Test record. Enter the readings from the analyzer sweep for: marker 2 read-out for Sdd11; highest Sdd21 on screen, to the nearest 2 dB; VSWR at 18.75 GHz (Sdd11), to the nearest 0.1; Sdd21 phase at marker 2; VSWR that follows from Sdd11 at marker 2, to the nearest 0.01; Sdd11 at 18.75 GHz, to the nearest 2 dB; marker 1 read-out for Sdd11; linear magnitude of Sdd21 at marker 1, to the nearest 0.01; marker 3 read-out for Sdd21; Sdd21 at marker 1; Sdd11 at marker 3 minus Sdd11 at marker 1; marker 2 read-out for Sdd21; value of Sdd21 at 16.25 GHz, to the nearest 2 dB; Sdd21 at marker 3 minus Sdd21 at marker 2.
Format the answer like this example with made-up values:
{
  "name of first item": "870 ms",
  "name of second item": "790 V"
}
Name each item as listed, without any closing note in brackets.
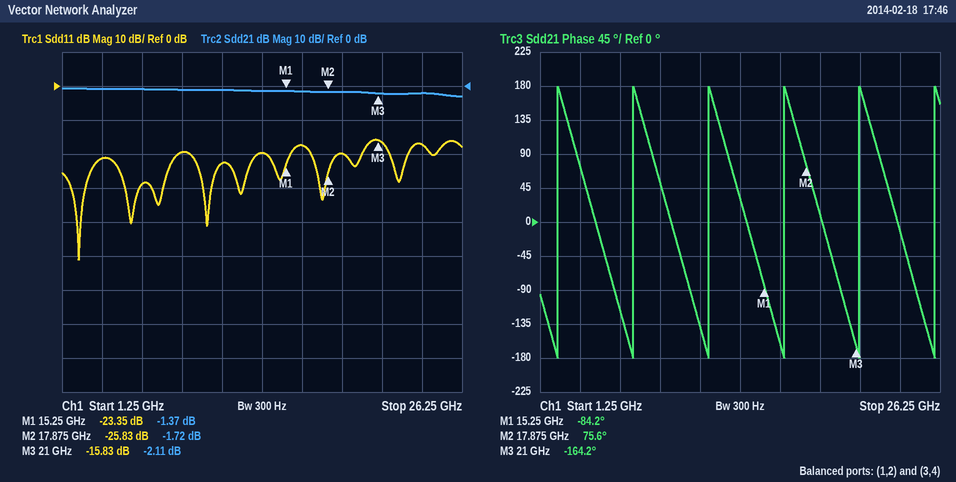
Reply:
{
  "marker 2 read-out for Sdd11": "-25.83 dB",
  "highest Sdd21 on screen, to the nearest 2 dB": "0 dB",
  "VSWR at 18.75 GHz (Sdd11), to the nearest 0.1": "1.2",
  "Sdd21 phase at marker 2": "75.6°",
  "VSWR that follows from Sdd11 at marker 2, to the nearest 0.01": "1.11",
  "Sdd11 at 18.75 GHz, to the nearest 2 dB": "-20 dB",
  "marker 1 read-out for Sdd11": "-23.35 dB",
  "linear magnitude of Sdd21 at marker 1, to the nearest 0.01": "0.85",
  "marker 3 read-out for Sdd21": "-2.11 dB",
  "Sdd21 at marker 1": "-1.37 dB",
  "Sdd11 at marker 3 minus Sdd11 at marker 1": "7.52 dB",
  "marker 2 read-out for Sdd21": "-1.72 dB",
  "value of Sdd21 at 16.25 GHz, to the nearest 2 dB": "-2 dB",
  "Sdd21 at marker 3 minus Sdd21 at marker 2": "-0.39 dB"
}
